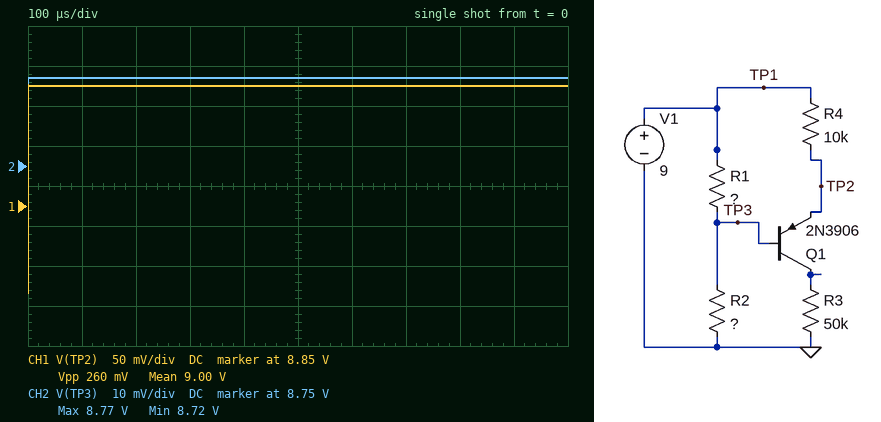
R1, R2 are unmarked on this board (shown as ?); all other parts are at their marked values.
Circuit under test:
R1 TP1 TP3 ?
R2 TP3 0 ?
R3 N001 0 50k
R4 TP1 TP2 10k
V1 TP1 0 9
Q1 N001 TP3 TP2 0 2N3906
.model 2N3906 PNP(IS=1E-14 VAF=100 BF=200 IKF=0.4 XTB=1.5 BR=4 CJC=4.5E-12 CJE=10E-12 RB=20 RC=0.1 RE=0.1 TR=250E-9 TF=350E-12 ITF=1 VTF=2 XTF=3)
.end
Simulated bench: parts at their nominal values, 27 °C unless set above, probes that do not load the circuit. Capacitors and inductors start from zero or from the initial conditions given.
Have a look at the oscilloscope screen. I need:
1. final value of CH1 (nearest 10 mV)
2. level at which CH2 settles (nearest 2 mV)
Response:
9.00 V
8.772 V
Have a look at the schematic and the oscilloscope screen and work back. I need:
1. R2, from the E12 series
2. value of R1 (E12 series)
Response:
15 kΩ
390 Ω
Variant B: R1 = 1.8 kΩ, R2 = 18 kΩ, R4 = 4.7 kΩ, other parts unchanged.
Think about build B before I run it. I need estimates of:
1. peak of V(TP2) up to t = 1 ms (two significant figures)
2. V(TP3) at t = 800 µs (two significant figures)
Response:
8.8 V
8.2 V
